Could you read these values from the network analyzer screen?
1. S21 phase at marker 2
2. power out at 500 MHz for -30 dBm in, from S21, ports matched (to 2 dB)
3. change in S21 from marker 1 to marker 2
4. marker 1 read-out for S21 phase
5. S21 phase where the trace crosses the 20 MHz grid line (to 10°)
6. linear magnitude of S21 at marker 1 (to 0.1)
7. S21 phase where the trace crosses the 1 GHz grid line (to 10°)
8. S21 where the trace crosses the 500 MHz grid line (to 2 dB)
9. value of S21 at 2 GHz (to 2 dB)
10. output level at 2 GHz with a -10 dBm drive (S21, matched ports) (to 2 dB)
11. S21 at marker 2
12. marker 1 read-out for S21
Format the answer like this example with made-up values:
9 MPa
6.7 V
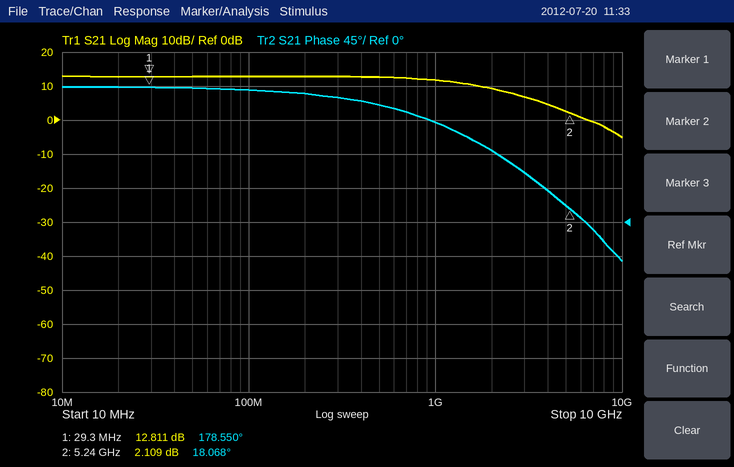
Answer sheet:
18.068°
-18 dBm
-10.702 dB
178.550°
180°
4.4
130°
12 dB
10 dB
0 dBm
2.109 dB
12.811 dB
